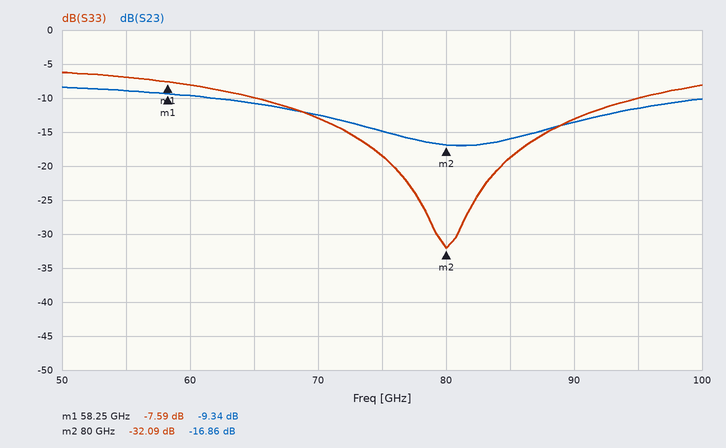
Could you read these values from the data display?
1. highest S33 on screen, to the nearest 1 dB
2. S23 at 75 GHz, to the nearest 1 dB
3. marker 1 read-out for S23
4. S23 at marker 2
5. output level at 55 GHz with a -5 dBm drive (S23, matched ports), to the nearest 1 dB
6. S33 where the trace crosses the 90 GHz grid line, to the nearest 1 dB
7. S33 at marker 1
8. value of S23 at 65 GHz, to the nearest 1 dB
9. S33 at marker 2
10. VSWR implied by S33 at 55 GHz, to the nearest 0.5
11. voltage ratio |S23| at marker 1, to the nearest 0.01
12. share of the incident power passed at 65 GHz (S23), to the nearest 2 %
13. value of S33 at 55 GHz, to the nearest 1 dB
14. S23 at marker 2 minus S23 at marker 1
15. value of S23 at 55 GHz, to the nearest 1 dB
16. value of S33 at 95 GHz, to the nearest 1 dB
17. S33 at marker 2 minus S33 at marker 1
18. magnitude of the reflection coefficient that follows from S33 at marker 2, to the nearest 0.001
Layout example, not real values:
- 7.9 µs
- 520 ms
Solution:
- -6 dB
- -15 dB
- -9.34 dB
- -16.86 dB
- -14 dBm
- -13 dB
- -7.59 dB
- -11 dB
- -32.09 dB
- 2.5
- 0.34
- 8 %
- -7 dB
- -7.52 dB
- -9 dB
- -10 dB
- -24.50 dB
- 0.025
